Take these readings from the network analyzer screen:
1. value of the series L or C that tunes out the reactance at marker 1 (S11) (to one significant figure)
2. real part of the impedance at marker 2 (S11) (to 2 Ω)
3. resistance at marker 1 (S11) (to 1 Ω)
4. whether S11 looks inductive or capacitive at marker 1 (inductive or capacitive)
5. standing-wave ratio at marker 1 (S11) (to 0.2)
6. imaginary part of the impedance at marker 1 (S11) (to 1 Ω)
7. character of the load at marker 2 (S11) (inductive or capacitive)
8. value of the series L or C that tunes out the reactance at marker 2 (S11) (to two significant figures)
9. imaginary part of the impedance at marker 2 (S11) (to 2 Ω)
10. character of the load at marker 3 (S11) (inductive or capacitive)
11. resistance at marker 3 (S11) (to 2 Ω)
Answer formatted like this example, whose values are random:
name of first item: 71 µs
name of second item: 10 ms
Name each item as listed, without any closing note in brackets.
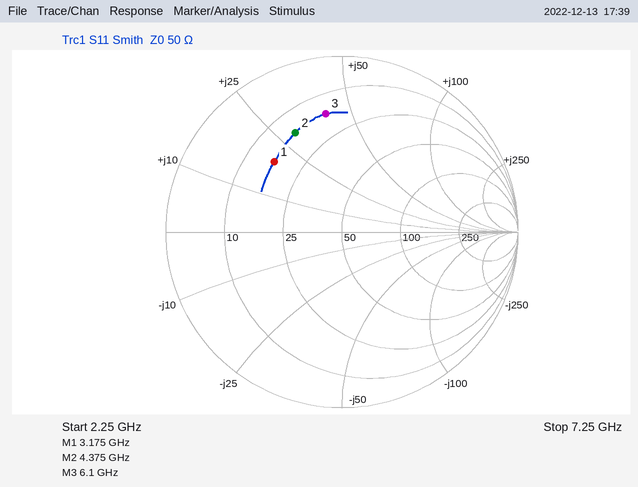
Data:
value of the series L or C that tunes out the reactance at marker 1 (S11): 3 pF
real part of the impedance at marker 2 (S11): 16 Ω
resistance at marker 1 (S11): 17 Ω
whether S11 looks inductive or capacitive at marker 1: inductive
standing-wave ratio at marker 1 (S11): 3.4
imaginary part of the impedance at marker 1 (S11): +19 Ω
character of the load at marker 2 (S11): inductive
value of the series L or C that tunes out the reactance at marker 2 (S11): 1.2 pF
imaginary part of the impedance at marker 2 (S11): +30 Ω
character of the load at marker 3 (S11): inductive
resistance at marker 3 (S11): 16 Ω
